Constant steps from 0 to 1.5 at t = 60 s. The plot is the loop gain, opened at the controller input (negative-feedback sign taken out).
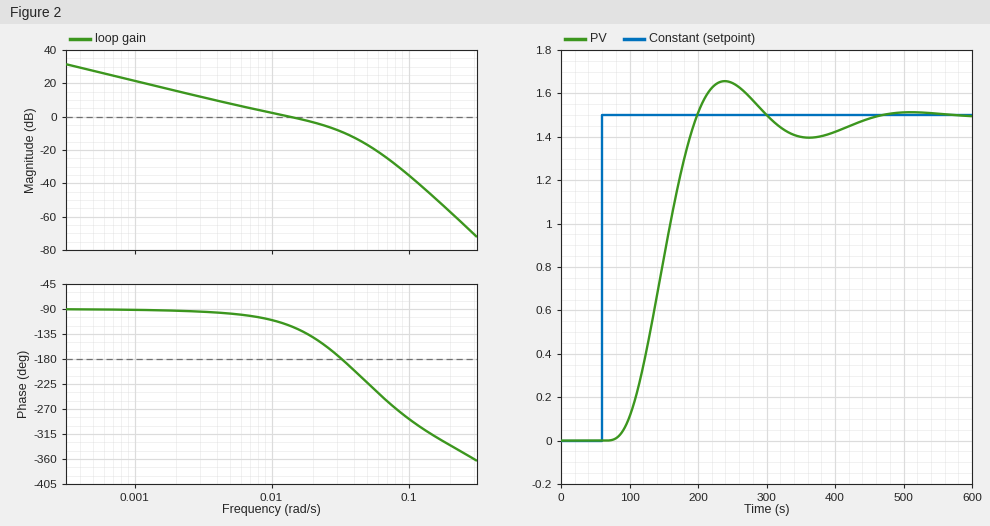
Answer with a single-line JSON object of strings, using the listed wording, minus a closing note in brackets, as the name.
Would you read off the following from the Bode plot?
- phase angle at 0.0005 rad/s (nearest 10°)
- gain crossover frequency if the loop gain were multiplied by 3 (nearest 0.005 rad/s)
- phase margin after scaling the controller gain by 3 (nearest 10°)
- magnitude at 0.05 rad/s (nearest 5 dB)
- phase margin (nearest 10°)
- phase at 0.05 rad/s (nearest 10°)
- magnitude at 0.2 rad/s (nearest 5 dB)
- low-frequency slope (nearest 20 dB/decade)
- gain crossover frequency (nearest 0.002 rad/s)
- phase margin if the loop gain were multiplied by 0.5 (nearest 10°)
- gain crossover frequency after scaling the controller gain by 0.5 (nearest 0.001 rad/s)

{"phase angle at 0.0005 rad/s": "-90°", "gain crossover frequency if the loop gain were multiplied by 3": "0.035 rad/s", "phase margin after scaling the controller gain by 3": "0°", "magnitude at 0.05 rad/s": "-15 dB", "phase margin": "60°", "phase at 0.05 rad/s": "-220°", "magnitude at 0.2 rad/s": "-55 dB", "low-frequency slope": "-20 dB/decade", "gain crossover frequency": "0.014 rad/s", "phase margin if the loop gain were multiplied by 0.5": "80°", "gain crossover frequency after scaling the controller gain by 0.5": "0.006 rad/s"}
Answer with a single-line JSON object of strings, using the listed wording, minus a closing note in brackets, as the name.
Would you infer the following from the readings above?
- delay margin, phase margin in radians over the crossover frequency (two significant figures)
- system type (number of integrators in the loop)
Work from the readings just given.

{"delay margin, phase margin in radians over the crossover frequency": "75 s", "system type": "1"}
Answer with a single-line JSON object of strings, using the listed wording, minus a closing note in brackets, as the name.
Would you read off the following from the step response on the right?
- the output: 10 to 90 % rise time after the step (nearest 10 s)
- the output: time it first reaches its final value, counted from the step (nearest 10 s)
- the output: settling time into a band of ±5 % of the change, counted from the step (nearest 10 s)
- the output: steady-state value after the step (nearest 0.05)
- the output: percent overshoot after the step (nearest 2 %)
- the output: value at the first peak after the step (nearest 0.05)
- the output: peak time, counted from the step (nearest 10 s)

{"the output: 10 to 90 % rise time after the step": "80 s", "the output: time it first reaches its final value, counted from the step": "140 s", "the output: settling time into a band of ±5 % of the change, counted from the step": "340 s", "the output: steady-state value after the step": "1.50", "the output: percent overshoot after the step": "10 %", "the output: value at the first peak after the step": "1.65", "the output: peak time, counted from the step": "180 s"}
